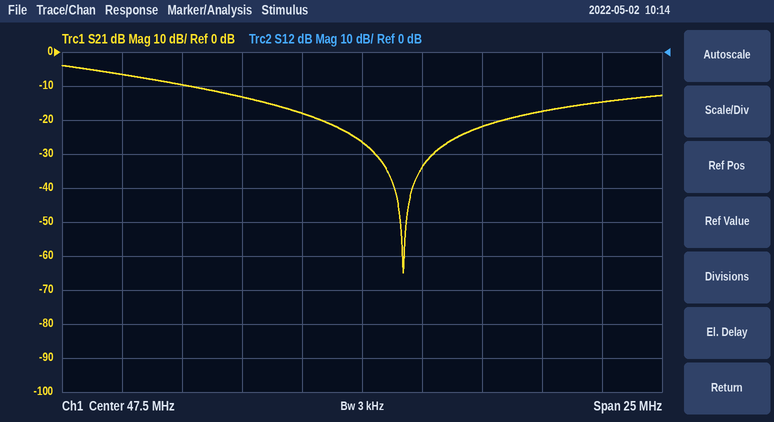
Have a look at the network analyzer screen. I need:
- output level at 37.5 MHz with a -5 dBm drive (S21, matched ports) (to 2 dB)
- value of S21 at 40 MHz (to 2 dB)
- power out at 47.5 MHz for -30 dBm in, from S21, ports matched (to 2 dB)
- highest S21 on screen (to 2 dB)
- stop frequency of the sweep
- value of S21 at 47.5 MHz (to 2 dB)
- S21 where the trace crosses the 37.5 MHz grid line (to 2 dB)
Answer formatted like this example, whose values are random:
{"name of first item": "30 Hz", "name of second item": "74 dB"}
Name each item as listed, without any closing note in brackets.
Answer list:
{"output level at 37.5 MHz with a -5 dBm drive (S21, matched ports)": "-12 dBm", "value of S21 at 40 MHz": "-10 dB", "power out at 47.5 MHz for -30 dBm in, from S21, ports matched": "-56 dBm", "highest S21 on screen": "-4 dB", "stop frequency of the sweep": "60 MHz", "value of S21 at 47.5 MHz": "-26 dB", "S21 where the trace crosses the 37.5 MHz grid line": "-6 dB"}
